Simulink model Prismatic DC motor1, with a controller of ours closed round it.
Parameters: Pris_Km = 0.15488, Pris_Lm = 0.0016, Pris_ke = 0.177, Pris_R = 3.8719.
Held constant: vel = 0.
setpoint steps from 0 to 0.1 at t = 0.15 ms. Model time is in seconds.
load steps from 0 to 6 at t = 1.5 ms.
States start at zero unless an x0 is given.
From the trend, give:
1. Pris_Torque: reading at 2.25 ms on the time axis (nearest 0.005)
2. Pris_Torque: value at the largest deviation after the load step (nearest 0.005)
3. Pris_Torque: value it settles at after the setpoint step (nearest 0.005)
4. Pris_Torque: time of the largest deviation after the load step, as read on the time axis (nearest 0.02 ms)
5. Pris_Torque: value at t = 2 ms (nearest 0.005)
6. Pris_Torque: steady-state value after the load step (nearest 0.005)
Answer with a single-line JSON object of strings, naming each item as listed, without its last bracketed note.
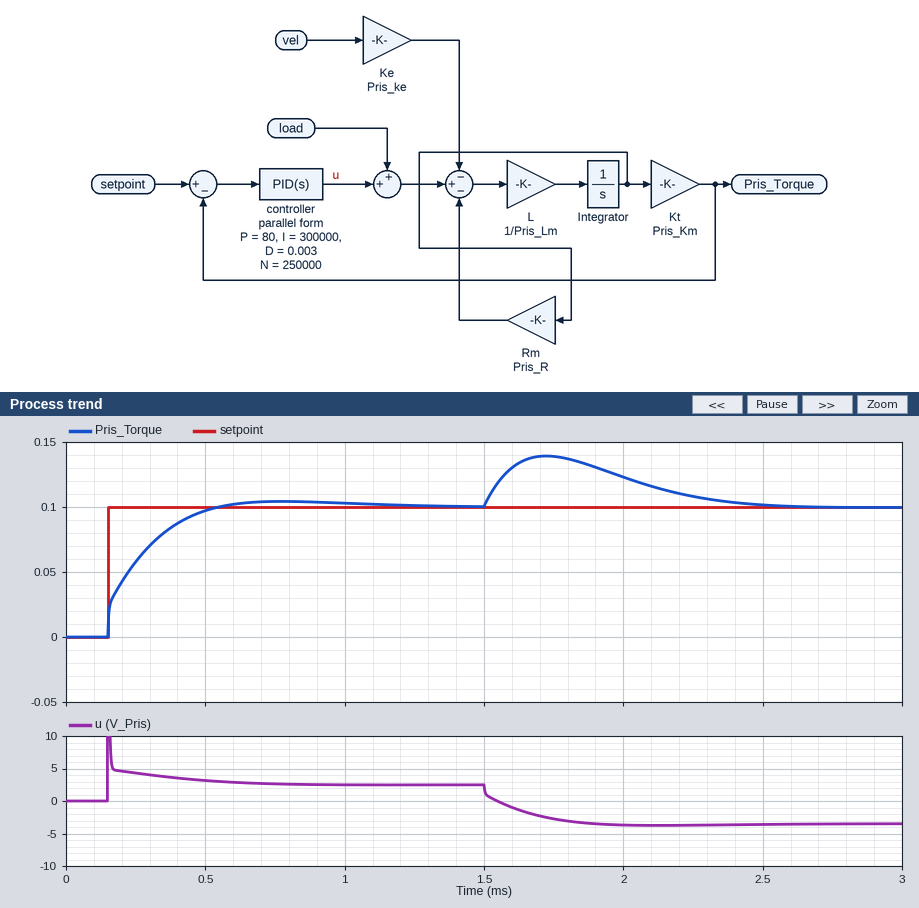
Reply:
{"Pris_Torque: reading at 2.25 ms on the time axis": "0.110", "Pris_Torque: value at the largest deviation after the load step": "0.140", "Pris_Torque: value it settles at after the setpoint step": "0.100", "Pris_Torque: time of the largest deviation after the load step, as read on the time axis": "1.72 ms", "Pris_Torque: value at t = 2 ms": "0.125", "Pris_Torque: steady-state value after the load step": "0.100"}
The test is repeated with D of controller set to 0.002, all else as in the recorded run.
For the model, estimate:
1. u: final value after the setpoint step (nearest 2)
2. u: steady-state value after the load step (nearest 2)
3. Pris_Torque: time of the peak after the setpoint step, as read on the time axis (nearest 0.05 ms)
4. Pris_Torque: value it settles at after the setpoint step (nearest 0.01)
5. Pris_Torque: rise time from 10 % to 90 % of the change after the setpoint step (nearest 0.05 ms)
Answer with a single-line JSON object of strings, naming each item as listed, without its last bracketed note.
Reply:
{"u: final value after the setpoint step": "2", "u: steady-state value after the load step": "-4", "Pris_Torque: time of the peak after the setpoint step, as read on the time axis": "0.75 ms", "Pris_Torque: value it settles at after the setpoint step": "0.10", "Pris_Torque: rise time from 10 % to 90 % of the change after the setpoint step": "0.25 ms"}
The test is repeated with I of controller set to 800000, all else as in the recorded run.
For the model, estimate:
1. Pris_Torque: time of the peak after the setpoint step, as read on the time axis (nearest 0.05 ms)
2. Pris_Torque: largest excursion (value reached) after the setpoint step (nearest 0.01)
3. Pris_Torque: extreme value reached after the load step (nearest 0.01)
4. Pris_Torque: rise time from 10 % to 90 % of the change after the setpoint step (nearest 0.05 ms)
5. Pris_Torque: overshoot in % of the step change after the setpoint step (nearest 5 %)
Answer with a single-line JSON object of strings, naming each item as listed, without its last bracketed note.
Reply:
{"Pris_Torque: time of the peak after the setpoint step, as read on the time axis": "0.50 ms", "Pris_Torque: largest excursion (value reached) after the setpoint step": "0.12", "Pris_Torque: extreme value reached after the load step": "0.13", "Pris_Torque: rise time from 10 % to 90 % of the change after the setpoint step": "0.15 ms", "Pris_Torque: overshoot in % of the step change after the setpoint step": "15 %"}
